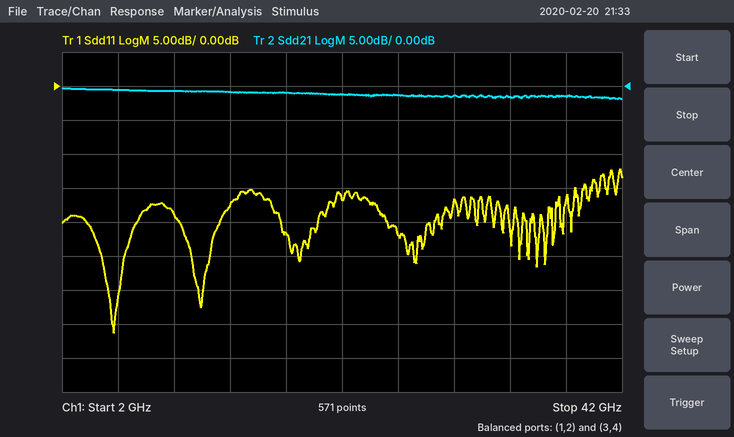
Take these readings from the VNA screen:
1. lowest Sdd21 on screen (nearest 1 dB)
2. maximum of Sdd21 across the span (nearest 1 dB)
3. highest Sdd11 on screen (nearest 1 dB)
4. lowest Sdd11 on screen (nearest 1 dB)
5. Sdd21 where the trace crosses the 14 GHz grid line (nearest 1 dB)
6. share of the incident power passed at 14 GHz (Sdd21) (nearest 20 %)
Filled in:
-2 dB
0 dB
-12 dB
-36 dB
-1 dB
80 %
